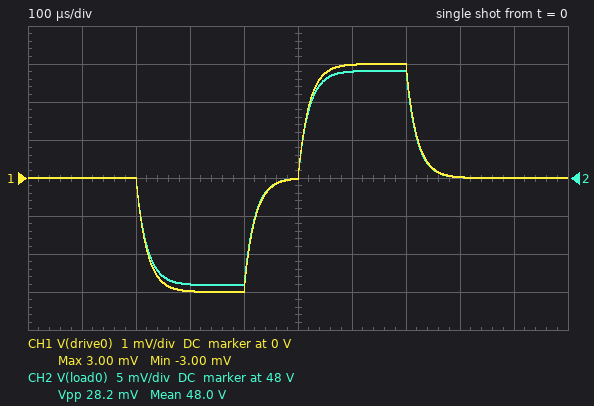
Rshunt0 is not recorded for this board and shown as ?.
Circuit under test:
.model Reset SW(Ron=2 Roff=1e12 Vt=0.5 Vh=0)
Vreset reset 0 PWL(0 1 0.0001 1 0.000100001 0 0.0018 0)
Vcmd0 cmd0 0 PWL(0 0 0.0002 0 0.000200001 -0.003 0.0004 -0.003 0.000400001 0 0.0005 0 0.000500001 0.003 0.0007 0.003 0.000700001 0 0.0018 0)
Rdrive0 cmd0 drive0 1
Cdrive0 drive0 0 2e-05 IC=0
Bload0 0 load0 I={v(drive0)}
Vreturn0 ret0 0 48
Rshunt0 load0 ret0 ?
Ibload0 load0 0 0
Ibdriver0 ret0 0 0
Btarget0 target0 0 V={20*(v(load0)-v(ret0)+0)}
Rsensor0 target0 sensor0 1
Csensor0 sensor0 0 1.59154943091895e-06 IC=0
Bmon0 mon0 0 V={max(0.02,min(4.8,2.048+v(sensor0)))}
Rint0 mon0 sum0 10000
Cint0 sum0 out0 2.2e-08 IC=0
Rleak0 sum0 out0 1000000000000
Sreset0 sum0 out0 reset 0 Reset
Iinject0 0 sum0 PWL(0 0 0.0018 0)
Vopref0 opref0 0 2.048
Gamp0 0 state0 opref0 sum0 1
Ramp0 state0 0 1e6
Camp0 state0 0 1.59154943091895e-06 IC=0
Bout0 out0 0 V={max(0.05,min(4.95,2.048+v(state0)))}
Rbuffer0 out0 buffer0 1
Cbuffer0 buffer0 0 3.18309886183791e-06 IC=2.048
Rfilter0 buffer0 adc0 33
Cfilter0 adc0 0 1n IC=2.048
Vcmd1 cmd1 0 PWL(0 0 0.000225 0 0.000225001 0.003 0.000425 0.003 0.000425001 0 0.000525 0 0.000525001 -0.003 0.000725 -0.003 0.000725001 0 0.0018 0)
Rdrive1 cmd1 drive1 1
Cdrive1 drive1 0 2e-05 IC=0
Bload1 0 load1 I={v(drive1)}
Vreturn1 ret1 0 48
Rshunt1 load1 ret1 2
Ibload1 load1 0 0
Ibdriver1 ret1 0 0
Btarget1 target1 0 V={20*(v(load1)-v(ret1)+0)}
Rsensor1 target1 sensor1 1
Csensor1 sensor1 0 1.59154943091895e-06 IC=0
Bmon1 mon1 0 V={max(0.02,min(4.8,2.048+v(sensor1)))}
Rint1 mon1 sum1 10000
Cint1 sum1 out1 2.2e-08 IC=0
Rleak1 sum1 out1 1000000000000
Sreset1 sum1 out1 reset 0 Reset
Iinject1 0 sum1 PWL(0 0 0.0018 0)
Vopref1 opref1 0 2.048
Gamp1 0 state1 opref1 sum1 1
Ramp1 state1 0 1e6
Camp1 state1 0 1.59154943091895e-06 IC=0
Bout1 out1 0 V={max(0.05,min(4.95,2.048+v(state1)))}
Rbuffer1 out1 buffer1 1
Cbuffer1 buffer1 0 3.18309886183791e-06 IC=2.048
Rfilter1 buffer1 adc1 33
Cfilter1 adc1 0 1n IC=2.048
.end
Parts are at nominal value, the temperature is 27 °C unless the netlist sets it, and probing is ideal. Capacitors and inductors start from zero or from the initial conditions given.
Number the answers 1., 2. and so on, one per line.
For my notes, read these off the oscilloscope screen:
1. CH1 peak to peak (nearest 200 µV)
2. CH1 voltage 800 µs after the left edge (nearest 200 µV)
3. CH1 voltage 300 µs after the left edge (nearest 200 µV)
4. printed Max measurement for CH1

1. 6.0 mV
2. 0 V
3. -3.0 mV
4. 3.00 mV
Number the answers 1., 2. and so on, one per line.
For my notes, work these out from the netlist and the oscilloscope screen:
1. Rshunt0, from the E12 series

1. 4.7 Ω
